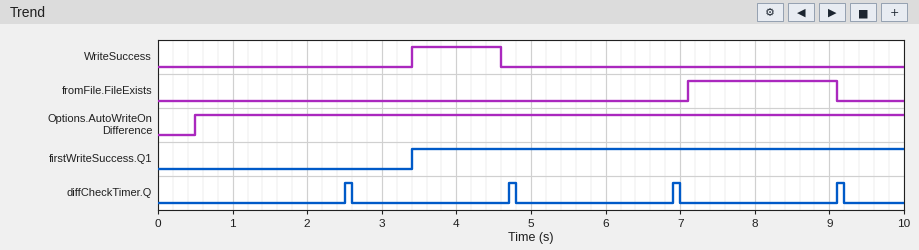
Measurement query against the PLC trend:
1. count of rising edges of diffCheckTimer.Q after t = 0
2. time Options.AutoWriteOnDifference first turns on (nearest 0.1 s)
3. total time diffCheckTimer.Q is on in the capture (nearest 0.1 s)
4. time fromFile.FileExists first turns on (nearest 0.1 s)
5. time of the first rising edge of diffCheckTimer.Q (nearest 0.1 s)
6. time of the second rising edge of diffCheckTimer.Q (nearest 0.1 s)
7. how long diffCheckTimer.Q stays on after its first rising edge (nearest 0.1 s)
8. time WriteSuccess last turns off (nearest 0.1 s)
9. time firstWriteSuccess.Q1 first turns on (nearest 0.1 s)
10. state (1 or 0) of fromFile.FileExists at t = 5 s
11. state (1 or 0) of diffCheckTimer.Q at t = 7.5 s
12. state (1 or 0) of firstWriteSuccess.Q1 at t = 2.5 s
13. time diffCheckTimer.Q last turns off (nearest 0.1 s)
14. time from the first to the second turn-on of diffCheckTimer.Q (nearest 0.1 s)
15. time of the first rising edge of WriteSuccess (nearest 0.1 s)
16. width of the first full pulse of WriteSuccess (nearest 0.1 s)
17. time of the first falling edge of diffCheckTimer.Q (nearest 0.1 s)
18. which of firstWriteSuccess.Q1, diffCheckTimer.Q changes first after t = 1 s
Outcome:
4
0.5 s
0.4 s
7.1 s
2.5 s
4.7 s
0.1 s
4.6 s
3.4 s
0
0
0
9.2 s
2.2 s
3.4 s
1.2 s
2.6 s
diffCheckTimer.Q
